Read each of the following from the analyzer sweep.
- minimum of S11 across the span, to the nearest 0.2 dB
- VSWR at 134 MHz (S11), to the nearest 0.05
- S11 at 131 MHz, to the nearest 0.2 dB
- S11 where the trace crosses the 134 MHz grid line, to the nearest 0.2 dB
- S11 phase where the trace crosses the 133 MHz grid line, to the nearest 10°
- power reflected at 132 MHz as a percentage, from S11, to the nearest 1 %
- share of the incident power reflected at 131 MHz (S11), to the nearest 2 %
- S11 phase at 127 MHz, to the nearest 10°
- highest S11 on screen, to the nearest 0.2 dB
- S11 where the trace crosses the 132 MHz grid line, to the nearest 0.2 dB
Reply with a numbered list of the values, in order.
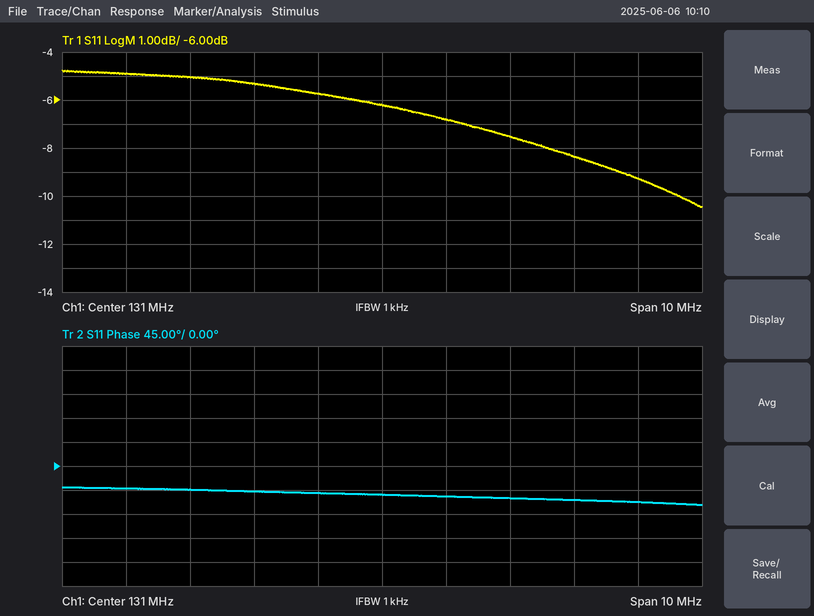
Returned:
1. -10.4 dB
2. 2.25
3. -6.2 dB
4. -8.4 dB
5. -60°
6. 21 %
7. 24 %
8. -40°
9. -4.8 dB
10. -6.8 dB
